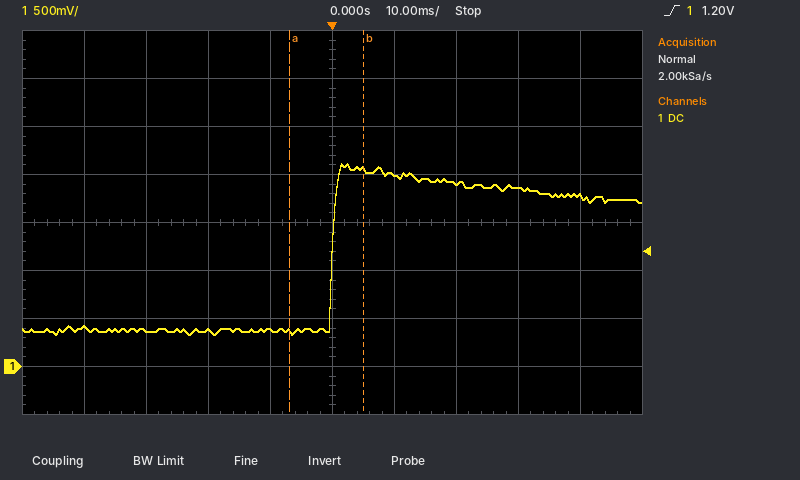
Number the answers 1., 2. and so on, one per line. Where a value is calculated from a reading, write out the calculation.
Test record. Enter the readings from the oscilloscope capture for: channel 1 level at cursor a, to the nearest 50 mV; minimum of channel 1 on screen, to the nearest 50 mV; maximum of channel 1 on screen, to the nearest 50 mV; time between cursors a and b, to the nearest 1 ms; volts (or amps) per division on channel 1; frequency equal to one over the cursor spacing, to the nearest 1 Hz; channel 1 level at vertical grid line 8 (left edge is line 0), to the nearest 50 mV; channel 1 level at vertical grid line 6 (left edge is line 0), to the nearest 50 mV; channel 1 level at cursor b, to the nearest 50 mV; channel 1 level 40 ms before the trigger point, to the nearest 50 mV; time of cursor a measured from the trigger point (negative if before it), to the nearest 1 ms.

1. 350 mV
2. 350 mV
3. 2.10 V
4. 12 ms
5. 500 mV
6. 1 / 12 ms ≈ 83 Hz
7. 1.85 V
8. 2.00 V
9. 2.05 V
10. 400 mV
11. -7 ms
